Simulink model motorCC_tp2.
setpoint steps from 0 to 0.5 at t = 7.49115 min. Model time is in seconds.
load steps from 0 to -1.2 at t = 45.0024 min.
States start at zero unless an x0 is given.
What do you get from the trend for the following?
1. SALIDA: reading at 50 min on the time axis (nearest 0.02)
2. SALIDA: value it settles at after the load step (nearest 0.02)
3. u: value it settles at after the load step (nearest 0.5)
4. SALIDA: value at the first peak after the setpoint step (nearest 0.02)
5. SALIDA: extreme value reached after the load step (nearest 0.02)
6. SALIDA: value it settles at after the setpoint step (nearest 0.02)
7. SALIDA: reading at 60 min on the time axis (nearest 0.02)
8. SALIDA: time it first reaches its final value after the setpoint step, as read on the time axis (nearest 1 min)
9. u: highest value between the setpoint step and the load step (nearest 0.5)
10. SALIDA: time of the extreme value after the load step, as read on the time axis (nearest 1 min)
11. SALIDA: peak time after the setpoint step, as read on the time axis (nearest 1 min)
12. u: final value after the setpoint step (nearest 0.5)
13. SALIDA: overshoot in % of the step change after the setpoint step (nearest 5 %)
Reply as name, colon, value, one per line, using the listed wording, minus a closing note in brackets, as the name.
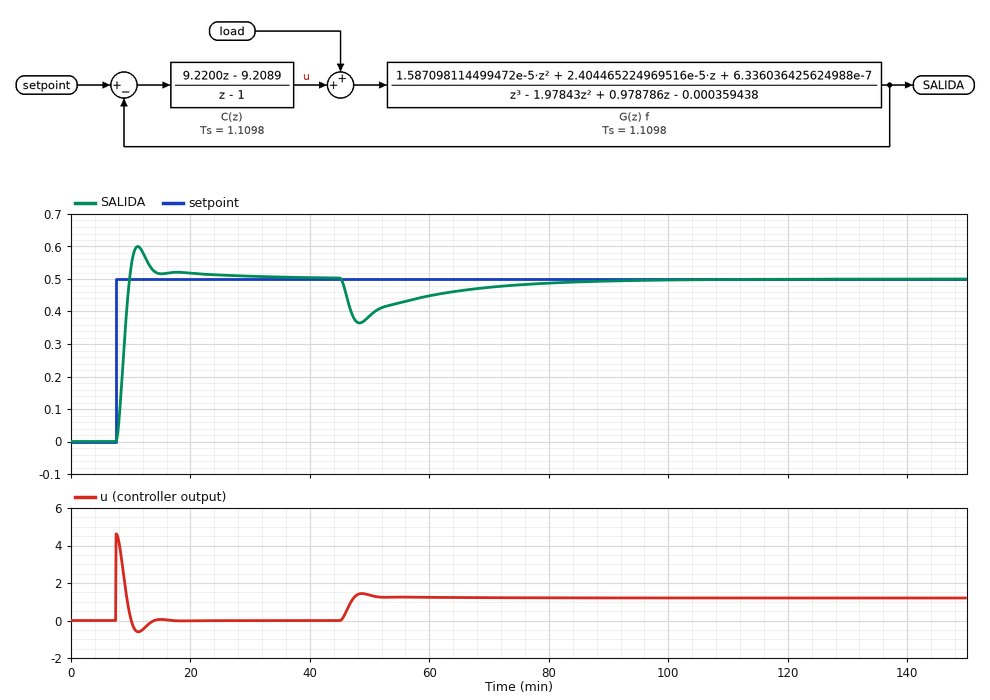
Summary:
SALIDA: reading at 50 min on the time axis: 0.38
SALIDA: value it settles at after the load step: 0.50
u: value it settles at after the load step: 1.0
SALIDA: value at the first peak after the setpoint step: 0.60
SALIDA: extreme value reached after the load step: 0.36
SALIDA: value it settles at after the setpoint step: 0.50
SALIDA: reading at 60 min on the time axis: 0.44
SALIDA: time it first reaches its final value after the setpoint step, as read on the time axis: 10 min
u: highest value between the setpoint step and the load step: 4.5
SALIDA: time of the extreme value after the load step, as read on the time axis: 48 min
SALIDA: peak time after the setpoint step, as read on the time axis: 11 min
u: final value after the setpoint step: 0.0
SALIDA: overshoot in % of the step change after the setpoint step: 20 %
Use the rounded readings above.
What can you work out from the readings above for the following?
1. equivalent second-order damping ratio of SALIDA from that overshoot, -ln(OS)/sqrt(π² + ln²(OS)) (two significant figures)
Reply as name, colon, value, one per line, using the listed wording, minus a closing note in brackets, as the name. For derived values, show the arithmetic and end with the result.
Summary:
equivalent second-order damping ratio of SALIDA from that overshoot, -ln(OS)/sqrt(π² + ln²(OS)): ln(0.2) = -1.609; 1.609 / sqrt(9.870 + 2.590) = 0.46
